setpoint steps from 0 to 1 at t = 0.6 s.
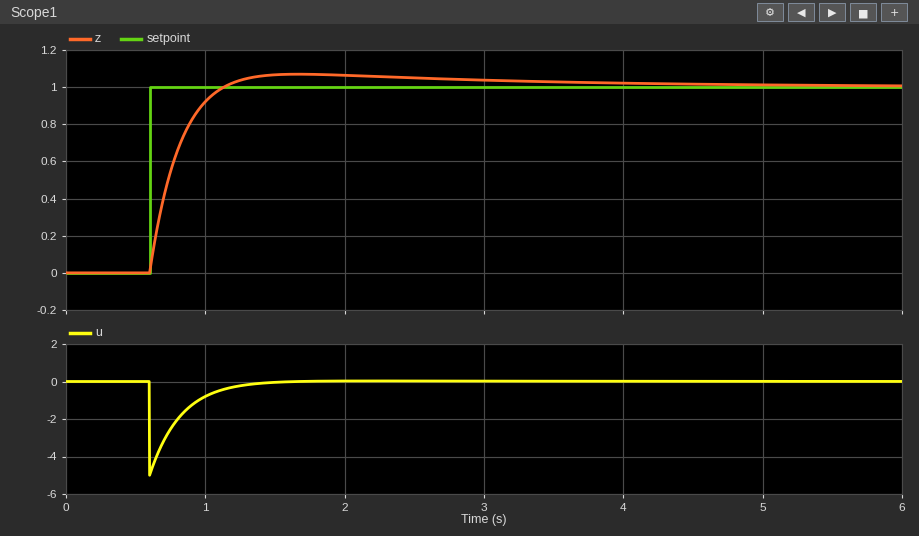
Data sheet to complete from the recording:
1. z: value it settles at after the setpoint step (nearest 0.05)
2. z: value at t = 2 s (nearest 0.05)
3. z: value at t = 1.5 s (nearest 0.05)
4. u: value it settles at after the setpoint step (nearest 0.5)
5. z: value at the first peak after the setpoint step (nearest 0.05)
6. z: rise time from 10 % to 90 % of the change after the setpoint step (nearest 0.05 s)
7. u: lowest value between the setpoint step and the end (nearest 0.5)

1.00
1.05
1.05
0.0
1.05
0.35 s
-5.0
